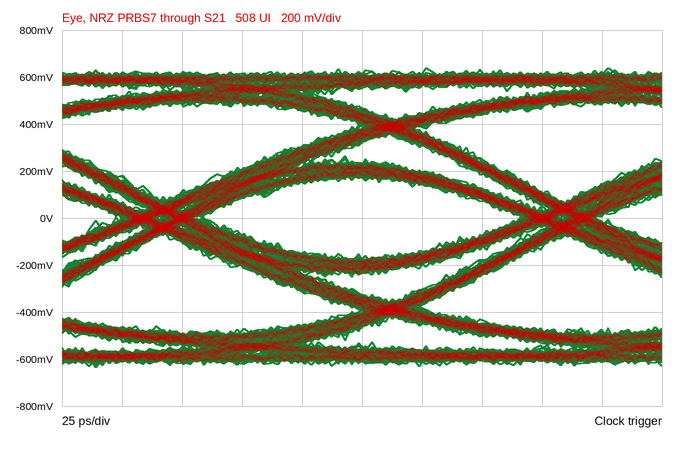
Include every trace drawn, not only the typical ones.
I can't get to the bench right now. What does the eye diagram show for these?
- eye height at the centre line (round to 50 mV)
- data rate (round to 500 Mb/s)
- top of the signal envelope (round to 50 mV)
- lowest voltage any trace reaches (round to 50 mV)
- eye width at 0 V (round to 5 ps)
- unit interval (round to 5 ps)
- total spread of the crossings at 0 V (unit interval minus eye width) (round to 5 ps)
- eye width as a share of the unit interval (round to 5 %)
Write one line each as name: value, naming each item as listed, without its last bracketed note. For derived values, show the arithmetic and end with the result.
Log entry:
eye height at the centre line: 350 mV
data rate: 6.0 Gb/s
top of the signal envelope: 650 mV
lowest voltage any trace reaches: -650 mV
eye width at 0 V: 130 ps
unit interval: 165 ps
total spread of the crossings at 0 V (unit interval minus eye width): 35 ps
eye width as a share of the unit interval: 130 ps / 165 ps ≈ 78.8 %, so 80 % to the nearest 5 %
